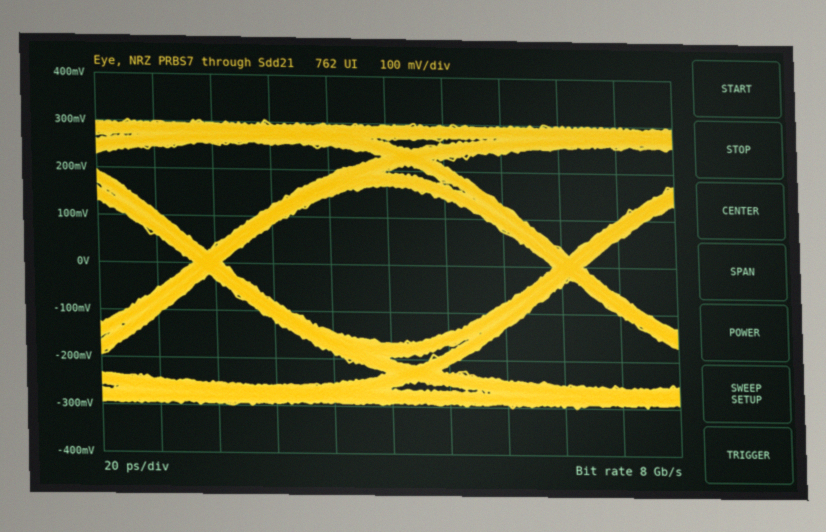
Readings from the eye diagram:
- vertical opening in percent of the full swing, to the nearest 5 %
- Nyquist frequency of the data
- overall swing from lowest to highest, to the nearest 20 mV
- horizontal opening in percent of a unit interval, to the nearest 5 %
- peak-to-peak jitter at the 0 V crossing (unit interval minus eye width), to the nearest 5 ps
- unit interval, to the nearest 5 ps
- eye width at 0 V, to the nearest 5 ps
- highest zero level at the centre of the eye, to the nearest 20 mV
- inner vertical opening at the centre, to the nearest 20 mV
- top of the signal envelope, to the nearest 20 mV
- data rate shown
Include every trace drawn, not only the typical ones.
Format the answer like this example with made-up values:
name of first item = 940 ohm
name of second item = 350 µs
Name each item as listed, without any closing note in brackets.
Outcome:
vertical opening in percent of the full swing, to the nearest 5 % = 55 %
Nyquist frequency of the data = 4 GHz
overall swing from lowest to highest, to the nearest 20 mV = 600 mV
horizontal opening in percent of a unit interval, to the nearest 5 % = 90 %
peak-to-peak jitter at the 0 V crossing (unit interval minus eye width), to the nearest 5 ps = 10 ps
unit interval, to the nearest 5 ps = 125 ps
eye width at 0 V, to the nearest 5 ps = 115 ps
highest zero level at the centre of the eye, to the nearest 20 mV = -160 mV
inner vertical opening at the centre, to the nearest 20 mV = 340 mV
top of the signal envelope, to the nearest 20 mV = 300 mV
data rate shown = 8 Gb/s
